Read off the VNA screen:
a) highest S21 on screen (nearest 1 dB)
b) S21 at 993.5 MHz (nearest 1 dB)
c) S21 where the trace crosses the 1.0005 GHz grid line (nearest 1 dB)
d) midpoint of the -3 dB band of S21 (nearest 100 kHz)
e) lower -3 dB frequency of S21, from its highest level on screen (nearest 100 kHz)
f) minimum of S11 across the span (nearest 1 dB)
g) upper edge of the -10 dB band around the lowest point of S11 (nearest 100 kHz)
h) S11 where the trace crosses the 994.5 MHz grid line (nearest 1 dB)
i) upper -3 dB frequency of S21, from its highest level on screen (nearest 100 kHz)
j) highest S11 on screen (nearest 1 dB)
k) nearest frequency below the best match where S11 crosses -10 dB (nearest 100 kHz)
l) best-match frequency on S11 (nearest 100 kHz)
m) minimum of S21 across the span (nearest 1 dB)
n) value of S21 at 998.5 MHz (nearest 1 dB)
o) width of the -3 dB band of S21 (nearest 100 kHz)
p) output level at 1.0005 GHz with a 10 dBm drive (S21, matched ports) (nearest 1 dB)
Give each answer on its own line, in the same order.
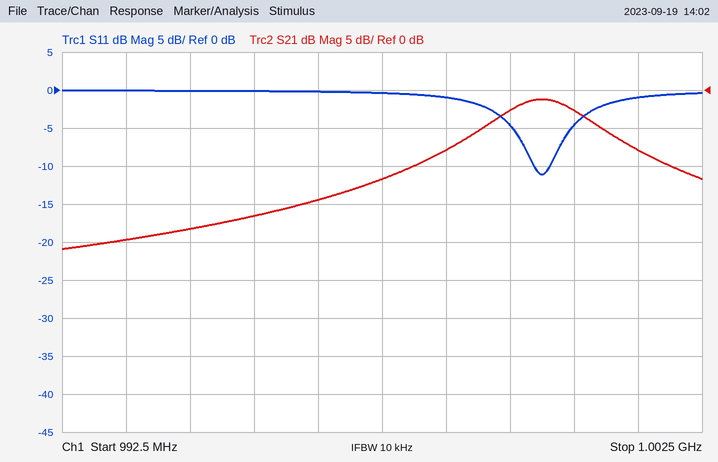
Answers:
-1 dB
-20 dB
-3 dB
1.0000 GHz
999.2 MHz
-11 dB
1.0001 GHz
0 dB
1.0008 GHz
0 dB
999.9 MHz
1.0000 GHz
-21 dB
-8 dB
1.6 MHz
7 dBm
